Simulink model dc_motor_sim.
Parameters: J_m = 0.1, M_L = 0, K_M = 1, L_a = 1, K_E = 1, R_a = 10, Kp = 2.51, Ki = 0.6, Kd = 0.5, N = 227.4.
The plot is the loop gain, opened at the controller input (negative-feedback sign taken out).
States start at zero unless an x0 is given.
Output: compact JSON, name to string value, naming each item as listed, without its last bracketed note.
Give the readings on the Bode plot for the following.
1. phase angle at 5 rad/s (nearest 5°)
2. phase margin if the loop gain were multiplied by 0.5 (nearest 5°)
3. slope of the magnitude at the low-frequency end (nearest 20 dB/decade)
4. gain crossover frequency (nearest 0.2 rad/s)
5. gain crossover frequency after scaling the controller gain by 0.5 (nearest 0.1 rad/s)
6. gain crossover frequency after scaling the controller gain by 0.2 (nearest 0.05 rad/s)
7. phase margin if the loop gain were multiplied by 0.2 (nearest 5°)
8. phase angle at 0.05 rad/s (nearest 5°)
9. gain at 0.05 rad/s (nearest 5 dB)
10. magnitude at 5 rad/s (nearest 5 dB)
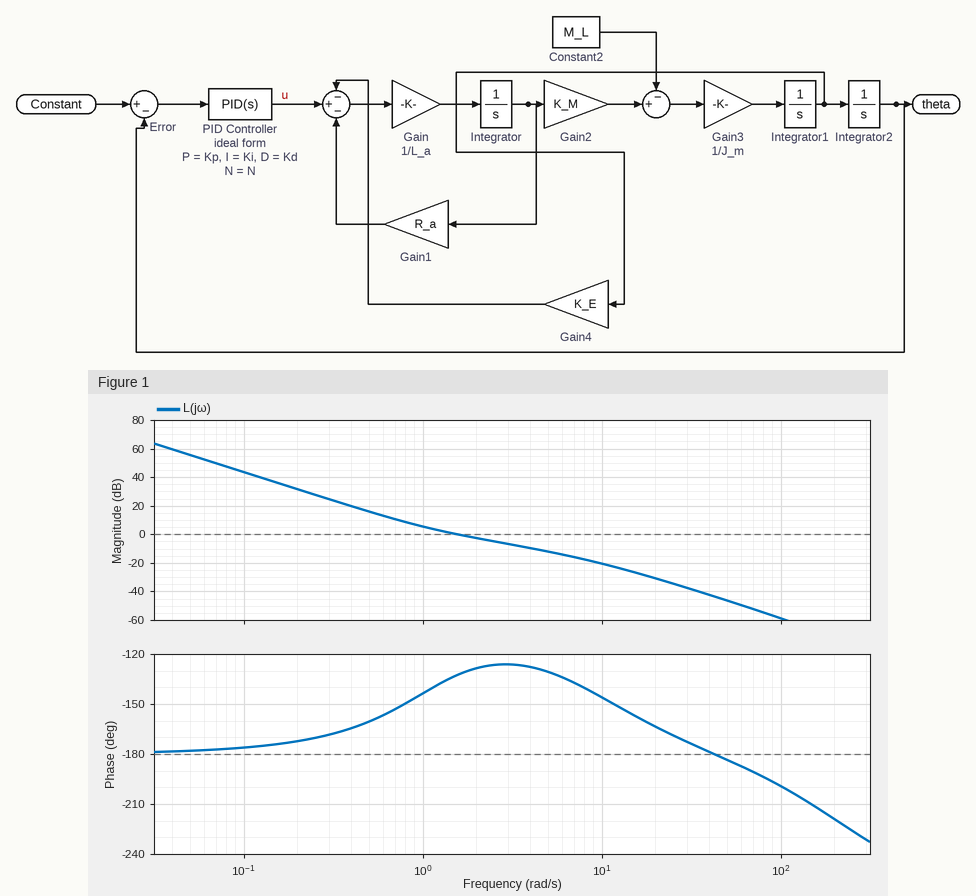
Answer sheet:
{"phase angle at 5 rad/s": "-130°", "phase margin if the loop gain were multiplied by 0.5": "35°", "slope of the magnitude at the low-frequency end": "-40 dB/decade", "gain crossover frequency": "1.6 rad/s", "gain crossover frequency after scaling the controller gain by 0.5": "1.0 rad/s", "gain crossover frequency after scaling the controller gain by 0.2": "0.55 rad/s", "phase margin if the loop gain were multiplied by 0.2": "20°", "phase angle at 0.05 rad/s": "-180°", "gain at 0.05 rad/s": "55 dB", "magnitude at 5 rad/s": "-10 dB"}
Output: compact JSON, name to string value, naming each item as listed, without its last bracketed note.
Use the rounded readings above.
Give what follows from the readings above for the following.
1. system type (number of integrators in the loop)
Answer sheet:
{"system type": "2"}
